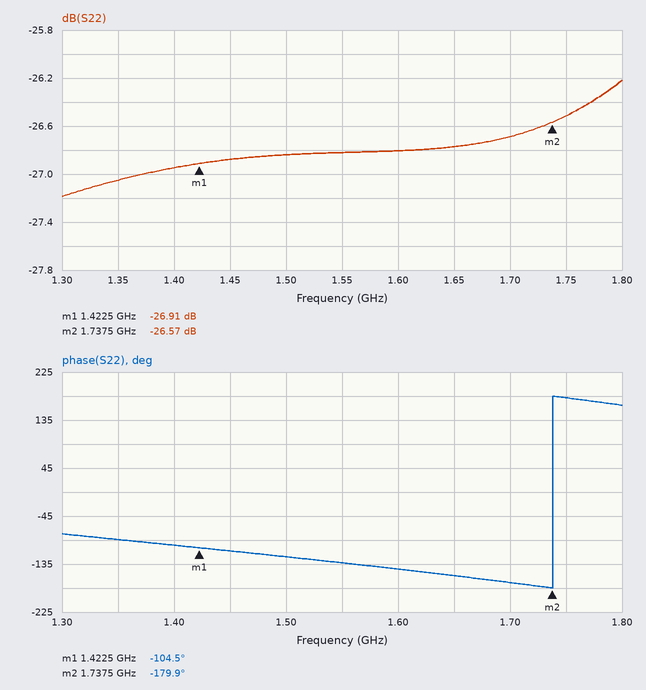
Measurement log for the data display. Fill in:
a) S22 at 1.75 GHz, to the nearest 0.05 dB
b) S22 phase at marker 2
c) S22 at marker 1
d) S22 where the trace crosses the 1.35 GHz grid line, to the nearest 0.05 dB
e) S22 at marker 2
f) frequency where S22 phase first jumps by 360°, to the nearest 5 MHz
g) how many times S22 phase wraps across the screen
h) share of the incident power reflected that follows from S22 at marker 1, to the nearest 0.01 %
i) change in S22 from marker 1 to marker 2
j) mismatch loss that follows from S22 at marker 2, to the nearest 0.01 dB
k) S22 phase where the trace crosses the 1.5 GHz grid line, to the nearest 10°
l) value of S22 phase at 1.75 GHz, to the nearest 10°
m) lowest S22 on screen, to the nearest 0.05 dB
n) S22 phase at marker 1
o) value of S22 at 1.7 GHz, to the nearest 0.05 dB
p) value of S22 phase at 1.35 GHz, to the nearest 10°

-26.50 dB
-179.9°
-26.91 dB
-27.05 dB
-26.57 dB
1.740 GHz
1
0.20 %
0.34 dB
0.01 dB
-120°
180°
-27.20 dB
-104.5°
-26.70 dB
-90°
